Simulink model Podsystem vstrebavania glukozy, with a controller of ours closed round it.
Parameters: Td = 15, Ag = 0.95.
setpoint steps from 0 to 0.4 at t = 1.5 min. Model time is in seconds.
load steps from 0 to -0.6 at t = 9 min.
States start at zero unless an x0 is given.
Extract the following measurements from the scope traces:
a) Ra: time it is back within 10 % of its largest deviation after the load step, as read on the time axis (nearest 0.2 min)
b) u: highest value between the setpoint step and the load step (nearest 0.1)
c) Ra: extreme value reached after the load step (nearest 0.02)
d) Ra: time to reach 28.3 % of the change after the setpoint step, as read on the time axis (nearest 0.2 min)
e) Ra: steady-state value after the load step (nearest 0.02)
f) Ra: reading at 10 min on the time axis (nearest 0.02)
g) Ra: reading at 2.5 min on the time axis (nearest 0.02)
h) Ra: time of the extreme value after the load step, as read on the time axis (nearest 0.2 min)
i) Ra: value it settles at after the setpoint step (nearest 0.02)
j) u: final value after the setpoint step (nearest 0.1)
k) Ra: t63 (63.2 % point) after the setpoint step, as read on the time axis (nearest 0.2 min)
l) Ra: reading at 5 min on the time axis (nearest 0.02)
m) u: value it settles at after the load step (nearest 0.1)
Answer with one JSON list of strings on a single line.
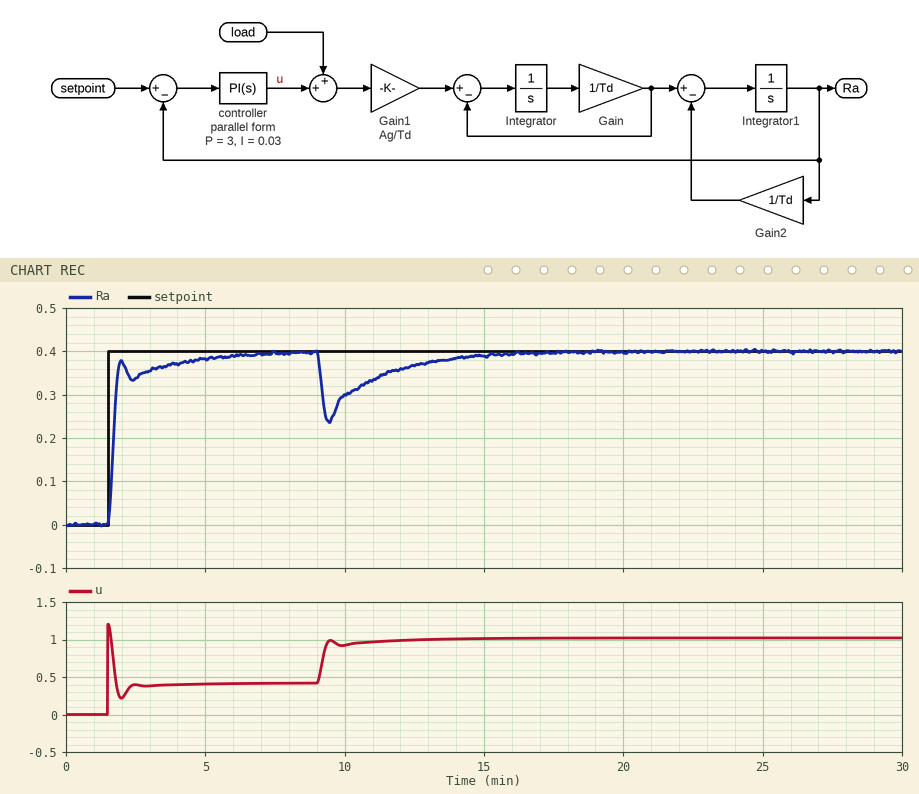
["14.0 min", "1.2", "0.24", "1.6 min", "0.40", "0.30", "0.34", "9.4 min", "0.40", "0.4", "1.8 min", "0.38", "1.0"]
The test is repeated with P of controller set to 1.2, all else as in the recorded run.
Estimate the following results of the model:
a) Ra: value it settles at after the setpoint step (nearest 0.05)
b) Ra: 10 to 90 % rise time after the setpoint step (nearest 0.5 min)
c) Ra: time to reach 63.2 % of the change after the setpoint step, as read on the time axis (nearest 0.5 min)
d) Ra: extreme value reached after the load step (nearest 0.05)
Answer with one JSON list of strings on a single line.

["0.40", "1.5 min", "2.0 min", "0.15"]
